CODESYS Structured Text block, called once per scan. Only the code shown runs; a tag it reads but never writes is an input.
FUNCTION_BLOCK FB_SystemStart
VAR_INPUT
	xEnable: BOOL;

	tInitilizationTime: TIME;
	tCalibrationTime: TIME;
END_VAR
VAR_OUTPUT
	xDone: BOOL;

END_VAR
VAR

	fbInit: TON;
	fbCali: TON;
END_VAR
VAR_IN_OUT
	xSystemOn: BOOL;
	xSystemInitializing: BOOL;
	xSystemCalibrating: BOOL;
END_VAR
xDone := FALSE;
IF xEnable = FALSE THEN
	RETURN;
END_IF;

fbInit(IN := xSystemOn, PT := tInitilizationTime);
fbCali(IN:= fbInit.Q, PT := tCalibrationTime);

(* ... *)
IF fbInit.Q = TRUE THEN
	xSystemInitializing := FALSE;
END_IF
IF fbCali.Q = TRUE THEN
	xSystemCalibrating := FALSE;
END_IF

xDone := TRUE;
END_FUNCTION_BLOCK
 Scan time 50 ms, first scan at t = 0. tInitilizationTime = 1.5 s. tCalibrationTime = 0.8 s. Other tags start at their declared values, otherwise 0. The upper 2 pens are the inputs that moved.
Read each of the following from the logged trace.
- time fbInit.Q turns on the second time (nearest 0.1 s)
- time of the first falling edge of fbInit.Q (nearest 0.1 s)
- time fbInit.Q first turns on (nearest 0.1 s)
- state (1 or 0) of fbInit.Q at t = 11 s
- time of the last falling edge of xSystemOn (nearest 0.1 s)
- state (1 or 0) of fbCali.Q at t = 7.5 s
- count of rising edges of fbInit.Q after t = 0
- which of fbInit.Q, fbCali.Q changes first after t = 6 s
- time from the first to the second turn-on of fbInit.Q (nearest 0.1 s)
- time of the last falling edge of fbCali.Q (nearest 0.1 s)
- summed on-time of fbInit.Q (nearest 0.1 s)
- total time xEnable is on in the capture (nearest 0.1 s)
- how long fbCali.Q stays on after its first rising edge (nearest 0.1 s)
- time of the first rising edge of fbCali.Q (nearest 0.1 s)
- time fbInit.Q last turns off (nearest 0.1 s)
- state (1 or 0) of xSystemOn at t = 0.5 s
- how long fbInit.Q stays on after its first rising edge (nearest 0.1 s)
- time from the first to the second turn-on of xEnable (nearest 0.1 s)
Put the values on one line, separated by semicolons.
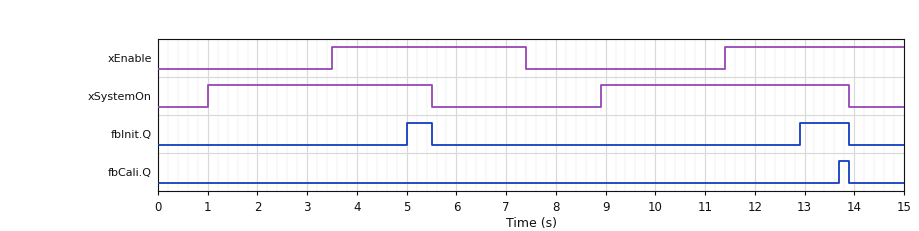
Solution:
12.9 s; 5.5 s; 5.0 s; 0; 13.9 s; 0; 2; fbInit.Q; 7.9 s; 13.9 s; 1.5 s; 7.5 s; 0.2 s; 13.7 s; 13.9 s; 0; 0.5 s; 7.9 s
